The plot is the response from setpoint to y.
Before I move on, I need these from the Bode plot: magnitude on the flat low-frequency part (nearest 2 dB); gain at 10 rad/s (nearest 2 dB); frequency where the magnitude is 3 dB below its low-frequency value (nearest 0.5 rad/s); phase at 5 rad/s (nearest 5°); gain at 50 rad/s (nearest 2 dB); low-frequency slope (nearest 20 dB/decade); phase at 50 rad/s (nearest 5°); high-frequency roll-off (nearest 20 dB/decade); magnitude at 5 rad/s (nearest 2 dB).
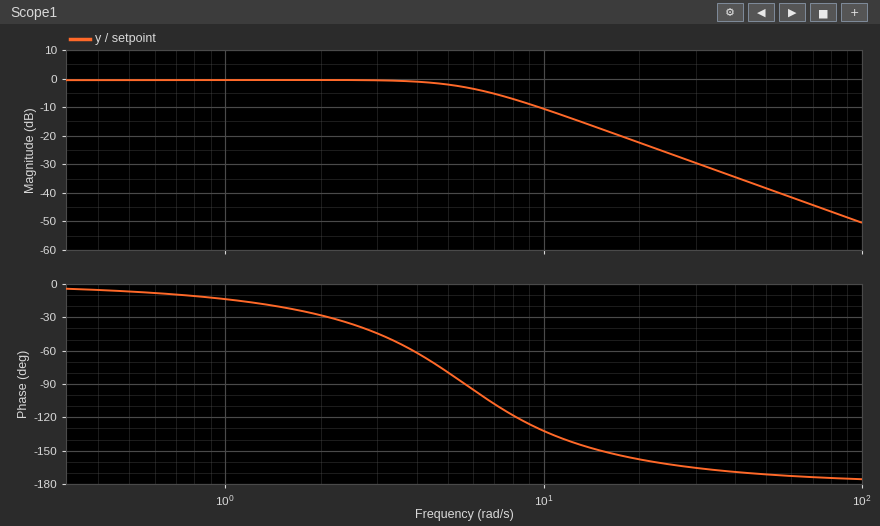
0 dB
-10 dB
6.0 rad/s
-80°
-38 dB
0 dB/decade
-170°
-40 dB/decade
-2 dB
